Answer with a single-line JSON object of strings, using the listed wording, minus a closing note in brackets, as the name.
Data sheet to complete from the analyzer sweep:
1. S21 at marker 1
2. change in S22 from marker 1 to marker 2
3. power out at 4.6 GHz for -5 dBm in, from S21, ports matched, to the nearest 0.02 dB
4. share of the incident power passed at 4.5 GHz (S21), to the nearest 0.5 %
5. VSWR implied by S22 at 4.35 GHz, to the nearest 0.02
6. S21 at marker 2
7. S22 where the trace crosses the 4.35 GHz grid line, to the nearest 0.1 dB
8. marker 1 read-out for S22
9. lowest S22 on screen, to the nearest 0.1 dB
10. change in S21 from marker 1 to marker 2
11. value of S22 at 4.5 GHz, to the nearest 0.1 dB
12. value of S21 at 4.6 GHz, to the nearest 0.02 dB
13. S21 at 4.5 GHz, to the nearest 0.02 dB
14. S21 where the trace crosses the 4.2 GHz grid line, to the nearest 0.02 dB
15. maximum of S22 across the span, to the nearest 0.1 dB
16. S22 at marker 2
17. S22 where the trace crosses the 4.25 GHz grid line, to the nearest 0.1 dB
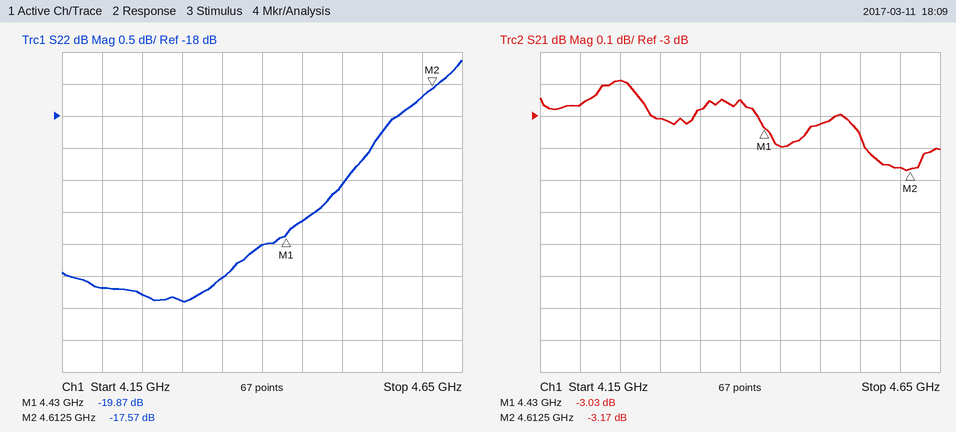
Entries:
{"S21 at marker 1": "-3.03 dB", "change in S22 from marker 1 to marker 2": "2.30 dB", "power out at 4.6 GHz for -5 dBm in, from S21, ports matched, to the nearest 0.02 dB": "-8.16 dBm", "share of the incident power passed at 4.5 GHz (S21), to the nearest 0.5 %": "50.0 %", "VSWR implied by S22 at 4.35 GHz, to the nearest 0.02": "1.20", "S21 at marker 2": "-3.17 dB", "S22 where the trace crosses the 4.35 GHz grid line, to the nearest 0.1 dB": "-20.5 dB", "marker 1 read-out for S22": "-19.87 dB", "lowest S22 on screen, to the nearest 0.1 dB": "-20.9 dB", "change in S21 from marker 1 to marker 2": "-0.14 dB", "value of S22 at 4.5 GHz, to the nearest 0.1 dB": "-19.1 dB", "value of S21 at 4.6 GHz, to the nearest 0.02 dB": "-3.16 dB", "S21 at 4.5 GHz, to the nearest 0.02 dB": "-3.02 dB", "S21 where the trace crosses the 4.2 GHz grid line, to the nearest 0.02 dB": "-2.96 dB", "maximum of S22 across the span, to the nearest 0.1 dB": "-17.1 dB", "S22 at marker 2": "-17.57 dB", "S22 where the trace crosses the 4.25 GHz grid line, to the nearest 0.1 dB": "-20.8 dB"}
